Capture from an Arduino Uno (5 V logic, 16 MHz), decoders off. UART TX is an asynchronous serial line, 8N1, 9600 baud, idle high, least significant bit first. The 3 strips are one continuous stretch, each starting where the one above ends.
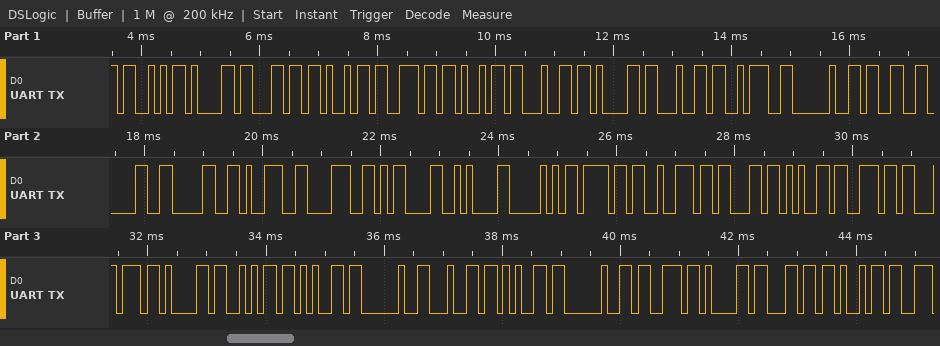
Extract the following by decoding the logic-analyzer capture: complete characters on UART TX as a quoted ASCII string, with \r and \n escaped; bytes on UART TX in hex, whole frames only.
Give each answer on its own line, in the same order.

"Salinidad: 30098\r\nPorcentaje de sali"
53 61 6C 69 6E 69 64 61 64 3A 20 33 30 30 39 38 0D 0A 50 6F 72 63 65 6E 74 61 6A 65 20 64 65 20 73 61 6C 69
